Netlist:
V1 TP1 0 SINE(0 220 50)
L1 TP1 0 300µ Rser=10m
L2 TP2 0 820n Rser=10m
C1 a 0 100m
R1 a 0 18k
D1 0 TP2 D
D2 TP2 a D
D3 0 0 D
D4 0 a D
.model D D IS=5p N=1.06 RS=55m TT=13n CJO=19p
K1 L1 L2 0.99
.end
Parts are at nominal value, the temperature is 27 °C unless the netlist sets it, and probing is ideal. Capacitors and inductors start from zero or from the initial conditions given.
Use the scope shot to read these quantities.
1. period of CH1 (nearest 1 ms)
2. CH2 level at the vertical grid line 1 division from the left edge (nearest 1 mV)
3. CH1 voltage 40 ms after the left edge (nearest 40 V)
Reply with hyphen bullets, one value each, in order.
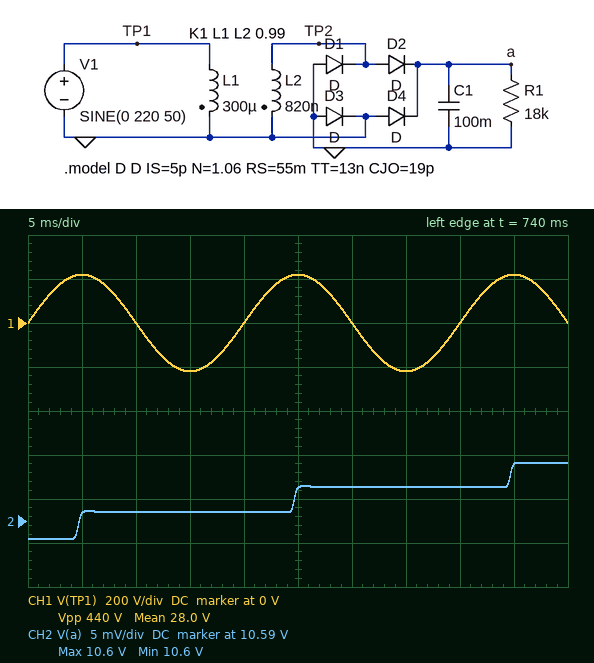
- 20 ms
- 10.586 V
- 0 V
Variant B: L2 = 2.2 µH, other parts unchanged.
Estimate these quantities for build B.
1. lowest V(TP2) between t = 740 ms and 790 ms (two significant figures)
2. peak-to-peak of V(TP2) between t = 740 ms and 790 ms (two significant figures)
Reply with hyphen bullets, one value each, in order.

- -16 V
- 34 V
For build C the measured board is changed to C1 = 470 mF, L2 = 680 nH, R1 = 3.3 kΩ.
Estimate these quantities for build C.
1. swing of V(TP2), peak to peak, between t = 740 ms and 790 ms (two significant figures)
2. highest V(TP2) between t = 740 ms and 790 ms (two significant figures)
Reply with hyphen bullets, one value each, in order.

- 19 V
- 10 V
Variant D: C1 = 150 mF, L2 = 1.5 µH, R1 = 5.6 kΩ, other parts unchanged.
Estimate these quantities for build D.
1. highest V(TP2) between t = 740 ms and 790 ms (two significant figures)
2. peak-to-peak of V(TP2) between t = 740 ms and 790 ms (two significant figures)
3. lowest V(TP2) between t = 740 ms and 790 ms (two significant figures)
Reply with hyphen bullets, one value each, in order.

- 15 V
- 28 V
- -13 V
